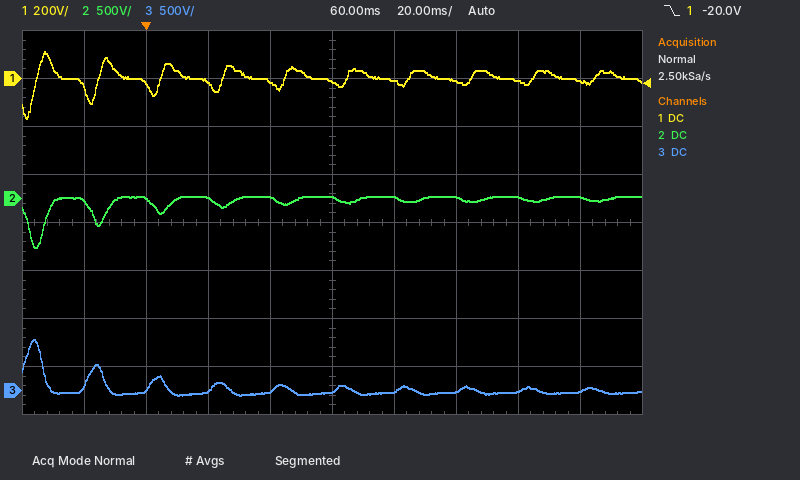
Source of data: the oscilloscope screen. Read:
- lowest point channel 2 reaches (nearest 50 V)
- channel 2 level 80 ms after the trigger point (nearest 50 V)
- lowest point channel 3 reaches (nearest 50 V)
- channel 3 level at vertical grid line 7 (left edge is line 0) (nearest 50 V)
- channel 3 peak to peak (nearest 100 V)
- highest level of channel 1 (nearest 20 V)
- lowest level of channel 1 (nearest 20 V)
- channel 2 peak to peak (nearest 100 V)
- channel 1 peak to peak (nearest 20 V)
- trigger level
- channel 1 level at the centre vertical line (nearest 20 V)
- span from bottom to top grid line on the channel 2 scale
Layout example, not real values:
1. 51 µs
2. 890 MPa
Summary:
1. -500 V
2. 0 V
3. -50 V
4. 0 V
5. 600 V
6. 120 V
7. -160 V
8. 500 V
9. 280 V
10. -20.0 V
11. -20 V
12. 4 kV
